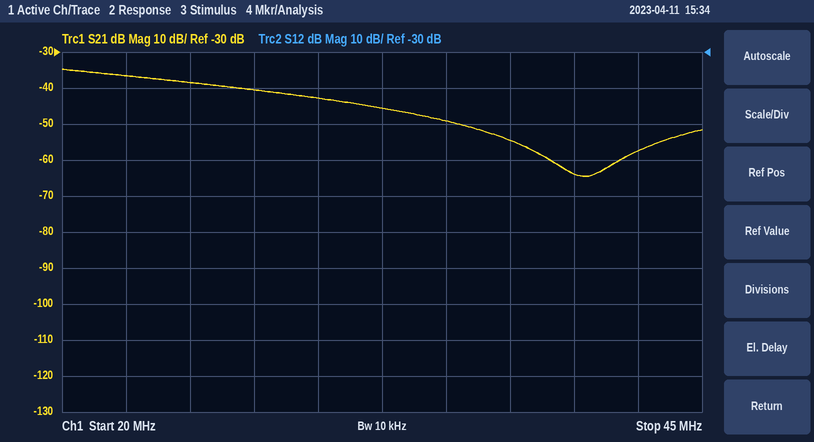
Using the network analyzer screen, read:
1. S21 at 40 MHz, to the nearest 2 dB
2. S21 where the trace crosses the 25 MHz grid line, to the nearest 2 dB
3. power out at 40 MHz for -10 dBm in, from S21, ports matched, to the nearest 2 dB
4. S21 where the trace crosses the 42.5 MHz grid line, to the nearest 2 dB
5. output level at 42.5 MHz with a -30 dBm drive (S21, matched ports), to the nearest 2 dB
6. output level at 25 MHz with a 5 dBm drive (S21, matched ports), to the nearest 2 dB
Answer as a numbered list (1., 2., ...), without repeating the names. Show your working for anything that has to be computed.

1. -64 dB
2. -38 dB
3. -10 dBm + (-64 dB) = -74 dBm
4. -58 dB
5. -30 dBm + (-58 dB) = -88 dBm
6. 5 dBm + (-38 dB) = -34 dBm
